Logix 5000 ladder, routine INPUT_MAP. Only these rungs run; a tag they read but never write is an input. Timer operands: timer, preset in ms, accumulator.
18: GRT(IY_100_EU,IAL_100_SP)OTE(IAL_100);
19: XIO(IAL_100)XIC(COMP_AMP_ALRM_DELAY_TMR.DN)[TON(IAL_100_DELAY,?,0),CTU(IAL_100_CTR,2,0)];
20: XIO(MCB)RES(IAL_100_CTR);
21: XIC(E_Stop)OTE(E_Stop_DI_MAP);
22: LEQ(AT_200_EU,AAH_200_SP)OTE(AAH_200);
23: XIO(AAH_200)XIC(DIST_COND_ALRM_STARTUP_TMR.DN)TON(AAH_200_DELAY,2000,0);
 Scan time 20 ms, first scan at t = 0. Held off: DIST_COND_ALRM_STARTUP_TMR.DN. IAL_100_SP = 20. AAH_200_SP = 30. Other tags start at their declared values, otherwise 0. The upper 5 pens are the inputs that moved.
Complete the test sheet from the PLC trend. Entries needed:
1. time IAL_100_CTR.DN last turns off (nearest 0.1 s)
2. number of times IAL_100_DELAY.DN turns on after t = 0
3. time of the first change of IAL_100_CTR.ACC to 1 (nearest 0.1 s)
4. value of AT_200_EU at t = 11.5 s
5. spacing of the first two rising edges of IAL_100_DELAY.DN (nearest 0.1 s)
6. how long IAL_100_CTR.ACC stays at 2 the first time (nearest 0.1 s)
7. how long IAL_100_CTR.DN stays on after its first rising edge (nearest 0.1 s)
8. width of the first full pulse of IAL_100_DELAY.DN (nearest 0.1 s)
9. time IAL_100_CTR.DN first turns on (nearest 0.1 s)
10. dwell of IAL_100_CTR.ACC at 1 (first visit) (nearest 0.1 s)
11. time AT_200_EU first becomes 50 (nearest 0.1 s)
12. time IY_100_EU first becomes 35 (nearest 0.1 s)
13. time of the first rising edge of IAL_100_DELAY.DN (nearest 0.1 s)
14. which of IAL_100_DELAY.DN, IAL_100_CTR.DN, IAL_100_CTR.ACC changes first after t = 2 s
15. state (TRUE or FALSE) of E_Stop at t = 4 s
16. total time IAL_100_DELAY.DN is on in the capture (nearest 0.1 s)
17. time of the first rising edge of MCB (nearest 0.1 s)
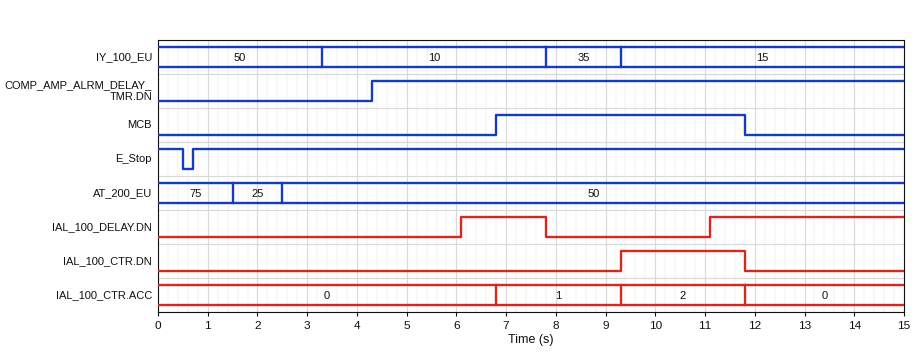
11.8 s
2
6.8 s
50
5.0 s
2.5 s
2.5 s
1.7 s
9.3 s
2.5 s
2.5 s
7.8 s
6.1 s
IAL_100_DELAY.DN
TRUE
5.6 s
6.8 s
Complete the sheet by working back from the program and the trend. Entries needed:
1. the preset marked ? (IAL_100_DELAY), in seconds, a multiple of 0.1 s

1.8 s
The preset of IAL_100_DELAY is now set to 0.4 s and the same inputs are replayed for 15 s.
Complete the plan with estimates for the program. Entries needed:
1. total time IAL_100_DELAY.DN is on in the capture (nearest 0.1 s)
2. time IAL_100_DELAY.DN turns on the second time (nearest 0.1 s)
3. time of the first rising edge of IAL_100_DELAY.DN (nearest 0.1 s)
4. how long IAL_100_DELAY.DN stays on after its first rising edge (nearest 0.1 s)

8.4 s
9.7 s
4.7 s
3.1 s
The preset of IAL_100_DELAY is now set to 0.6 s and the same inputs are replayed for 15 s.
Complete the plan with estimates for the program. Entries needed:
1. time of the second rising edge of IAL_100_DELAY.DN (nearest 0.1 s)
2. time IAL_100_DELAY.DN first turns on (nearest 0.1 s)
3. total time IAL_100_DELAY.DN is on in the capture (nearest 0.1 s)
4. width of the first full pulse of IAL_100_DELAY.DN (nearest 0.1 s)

9.9 s
4.9 s
8.0 s
2.9 s
